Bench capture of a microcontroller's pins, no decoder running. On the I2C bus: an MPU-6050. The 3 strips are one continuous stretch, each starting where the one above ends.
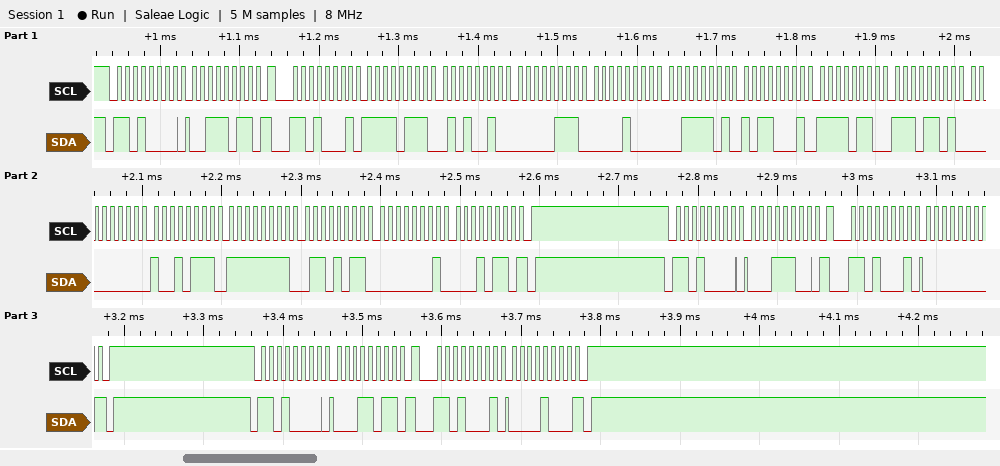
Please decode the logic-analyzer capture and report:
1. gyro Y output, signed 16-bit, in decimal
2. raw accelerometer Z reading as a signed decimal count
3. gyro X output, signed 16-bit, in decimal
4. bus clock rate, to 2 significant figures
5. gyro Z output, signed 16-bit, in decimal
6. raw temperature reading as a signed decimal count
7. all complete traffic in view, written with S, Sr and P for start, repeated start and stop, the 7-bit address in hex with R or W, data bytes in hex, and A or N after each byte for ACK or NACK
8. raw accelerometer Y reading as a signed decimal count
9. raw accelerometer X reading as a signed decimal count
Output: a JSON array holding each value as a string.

["-149", "15793", "151", "100 kHz", "278", "-2323", "S 68W A 3B A Sr 68R A F7 A 52 A 07 A 08 A 3D A B1 A F6 A ED A 00 A 97 A FF A 6B A 01 A 16 N P S 68W A 1C A Sr 68R A 00 N P S 68W A 1B A Sr 68R A 08 N P", "1800", "-2222"]
